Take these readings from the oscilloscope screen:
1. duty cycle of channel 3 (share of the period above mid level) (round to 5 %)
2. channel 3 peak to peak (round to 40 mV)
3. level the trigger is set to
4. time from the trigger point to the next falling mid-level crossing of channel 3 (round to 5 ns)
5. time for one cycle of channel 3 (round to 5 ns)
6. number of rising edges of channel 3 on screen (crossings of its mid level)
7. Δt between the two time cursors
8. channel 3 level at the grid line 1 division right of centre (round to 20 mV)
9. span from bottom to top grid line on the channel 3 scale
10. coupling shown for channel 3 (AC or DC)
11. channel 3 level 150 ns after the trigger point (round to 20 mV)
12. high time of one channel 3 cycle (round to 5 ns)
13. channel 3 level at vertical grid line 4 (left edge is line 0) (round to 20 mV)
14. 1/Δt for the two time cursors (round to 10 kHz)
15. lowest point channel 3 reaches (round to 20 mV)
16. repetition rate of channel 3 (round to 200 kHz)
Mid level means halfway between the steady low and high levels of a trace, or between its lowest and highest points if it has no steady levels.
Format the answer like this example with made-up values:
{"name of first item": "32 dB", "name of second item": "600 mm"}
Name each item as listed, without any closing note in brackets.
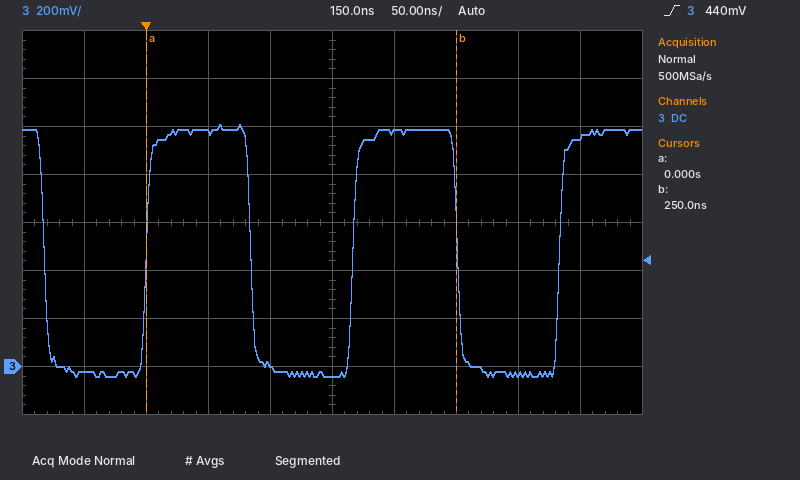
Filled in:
{"duty cycle of channel 3 (share of the period above mid level)": "50 %", "channel 3 peak to peak": "1.04 V", "level the trigger is set to": "440 mV", "time from the trigger point to the next falling mid-level crossing of channel 3": "85 ns", "time for one cycle of channel 3": "165 ns", "number of rising edges of channel 3 on screen": "3", "Δt between the two time cursors": "250 ns", "channel 3 level at the grid line 1 division right of centre": "980 mV", "span from bottom to top grid line on the channel 3 scale": "1.6 V", "coupling shown for channel 3": "DC", "channel 3 level 150 ns after the trigger point": "-40 mV", "high time of one channel 3 cycle": "85 ns", "channel 3 level at vertical grid line 4 (left edge is line 0)": "0 mV", "1/Δt for the two time cursors": "4.00 MHz", "lowest point channel 3 reaches": "-40 mV", "repetition rate of channel 3": "6.0 MHz"}
